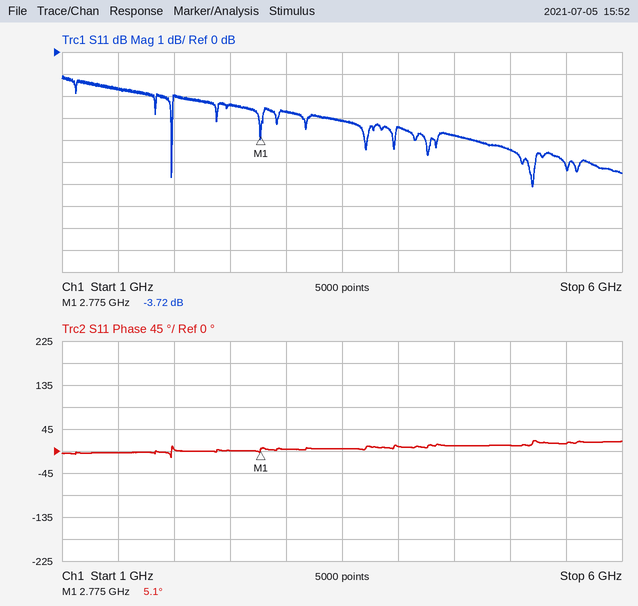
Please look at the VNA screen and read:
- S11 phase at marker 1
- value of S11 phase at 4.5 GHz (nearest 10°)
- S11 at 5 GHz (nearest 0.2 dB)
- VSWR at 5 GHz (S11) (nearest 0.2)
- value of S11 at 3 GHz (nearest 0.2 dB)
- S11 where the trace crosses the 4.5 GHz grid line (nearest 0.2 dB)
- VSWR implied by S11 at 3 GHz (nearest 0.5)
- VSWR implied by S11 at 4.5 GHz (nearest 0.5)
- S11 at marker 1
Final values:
5.1°
10°
-4.4 dB
4.0
-2.8 dB
-3.8 dB
6.5
4.5
-3.72 dB
